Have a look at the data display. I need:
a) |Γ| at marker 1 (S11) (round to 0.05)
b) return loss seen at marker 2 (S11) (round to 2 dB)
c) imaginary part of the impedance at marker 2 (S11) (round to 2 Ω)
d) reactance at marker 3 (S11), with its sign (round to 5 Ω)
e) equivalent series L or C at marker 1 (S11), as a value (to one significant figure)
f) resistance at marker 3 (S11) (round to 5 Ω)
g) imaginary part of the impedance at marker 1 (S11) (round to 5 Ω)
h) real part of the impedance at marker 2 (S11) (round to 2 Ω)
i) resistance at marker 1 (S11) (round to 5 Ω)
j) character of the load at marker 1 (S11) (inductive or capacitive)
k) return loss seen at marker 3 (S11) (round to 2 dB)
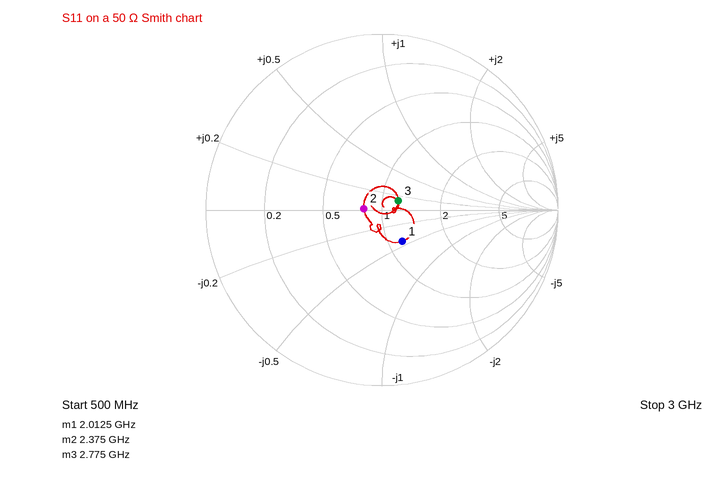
0.20
20 dB
0 Ω
+5 Ω
4 pF
60 Ω
-20 Ω
40 Ω
60 Ω
capacitive
20 dB
